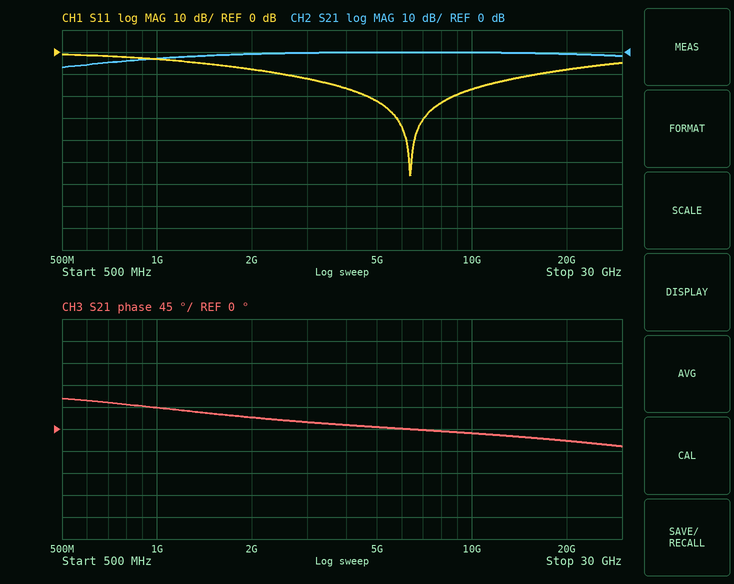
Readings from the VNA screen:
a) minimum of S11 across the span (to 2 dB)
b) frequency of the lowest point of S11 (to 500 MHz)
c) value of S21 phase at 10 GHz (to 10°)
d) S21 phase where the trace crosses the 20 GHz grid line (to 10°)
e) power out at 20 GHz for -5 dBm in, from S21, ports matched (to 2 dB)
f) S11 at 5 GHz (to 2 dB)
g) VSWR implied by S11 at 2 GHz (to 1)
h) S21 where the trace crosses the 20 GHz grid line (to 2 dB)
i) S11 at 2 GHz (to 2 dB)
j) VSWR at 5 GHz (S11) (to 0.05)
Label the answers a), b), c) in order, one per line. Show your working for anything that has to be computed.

a) -56 dB
b) 6.5 GHz
c) -10°
d) -20°
e) -5 dBm + (0 dB) = -6 dBm
f) -22 dB
g) |Γ| = 10^(-8/20) = 0.3981; VSWR = (1 + 0.3981)/(1 − 0.3981) ≈ 2
h) 0 dB
i) -8 dB
j) |Γ| = 10^(-22/20) = 0.0794; VSWR = (1 + 0.0794)/(1 − 0.0794) ≈ 1.17, so 1.15 to the nearest 0.05
